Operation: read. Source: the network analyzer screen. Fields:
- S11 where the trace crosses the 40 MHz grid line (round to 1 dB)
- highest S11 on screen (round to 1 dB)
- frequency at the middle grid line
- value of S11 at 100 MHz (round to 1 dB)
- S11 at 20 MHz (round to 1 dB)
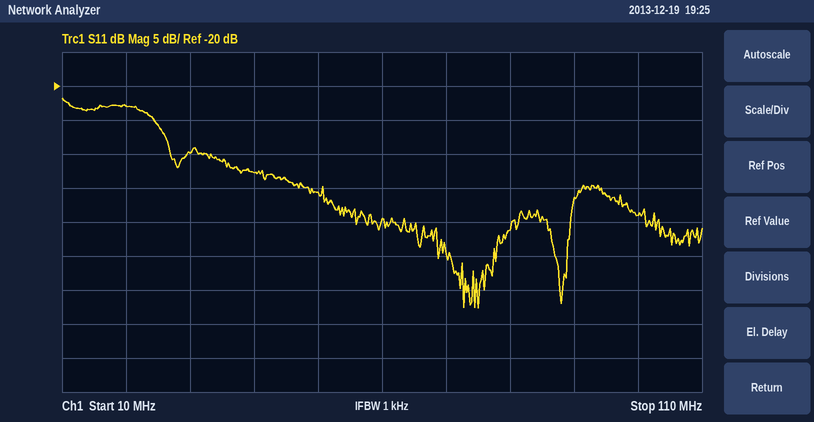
-33 dB
-22 dB
60 MHz
-39 dB
-23 dB
